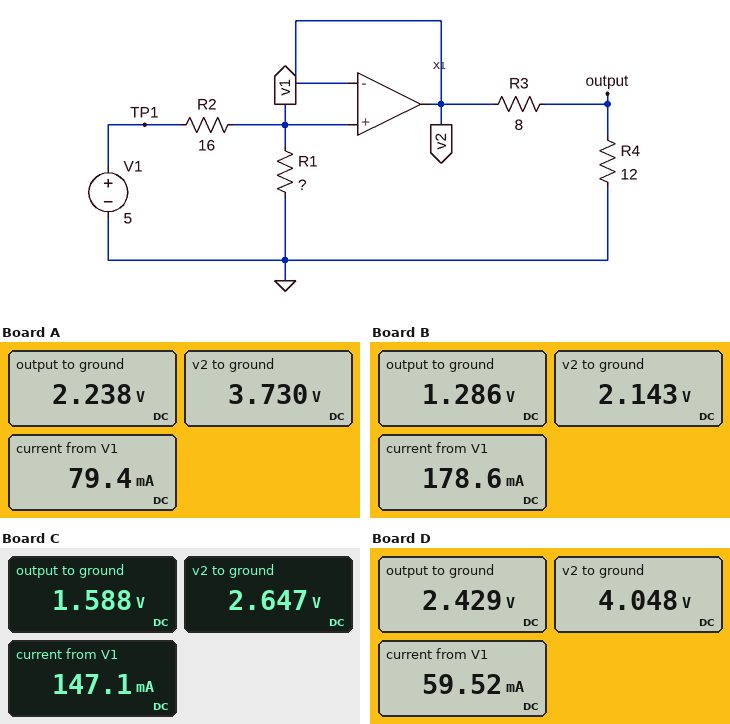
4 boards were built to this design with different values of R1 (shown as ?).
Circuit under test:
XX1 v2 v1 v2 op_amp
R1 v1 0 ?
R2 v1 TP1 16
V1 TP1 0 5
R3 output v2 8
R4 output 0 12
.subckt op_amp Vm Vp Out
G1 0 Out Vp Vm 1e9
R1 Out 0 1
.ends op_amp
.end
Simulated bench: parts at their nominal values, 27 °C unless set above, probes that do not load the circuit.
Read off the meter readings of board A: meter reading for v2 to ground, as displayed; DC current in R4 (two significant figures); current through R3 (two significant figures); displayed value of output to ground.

3.730 V
190 mA
190 mA
2.238 V
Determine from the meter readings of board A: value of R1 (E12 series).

47 Ω
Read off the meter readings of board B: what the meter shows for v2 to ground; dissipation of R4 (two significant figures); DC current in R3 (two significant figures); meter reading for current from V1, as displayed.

2.143 V
140 mW
110 mA
178.6 mA
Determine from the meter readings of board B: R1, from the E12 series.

12 Ω
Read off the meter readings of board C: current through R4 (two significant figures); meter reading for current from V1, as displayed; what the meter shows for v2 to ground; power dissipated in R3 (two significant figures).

130 mA
147.1 mA
2.647 V
140 mW
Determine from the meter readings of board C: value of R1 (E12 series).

18 Ω
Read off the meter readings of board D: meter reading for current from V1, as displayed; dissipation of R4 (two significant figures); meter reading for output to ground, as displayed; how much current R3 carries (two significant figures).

59.52 mA
490 mW
2.429 V
200 mA
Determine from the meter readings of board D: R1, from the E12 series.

68 Ω
